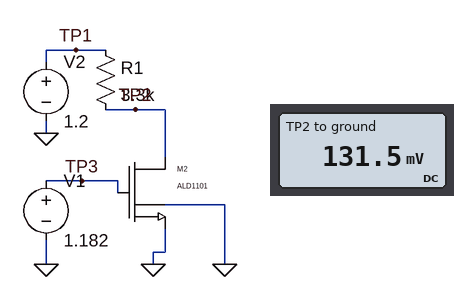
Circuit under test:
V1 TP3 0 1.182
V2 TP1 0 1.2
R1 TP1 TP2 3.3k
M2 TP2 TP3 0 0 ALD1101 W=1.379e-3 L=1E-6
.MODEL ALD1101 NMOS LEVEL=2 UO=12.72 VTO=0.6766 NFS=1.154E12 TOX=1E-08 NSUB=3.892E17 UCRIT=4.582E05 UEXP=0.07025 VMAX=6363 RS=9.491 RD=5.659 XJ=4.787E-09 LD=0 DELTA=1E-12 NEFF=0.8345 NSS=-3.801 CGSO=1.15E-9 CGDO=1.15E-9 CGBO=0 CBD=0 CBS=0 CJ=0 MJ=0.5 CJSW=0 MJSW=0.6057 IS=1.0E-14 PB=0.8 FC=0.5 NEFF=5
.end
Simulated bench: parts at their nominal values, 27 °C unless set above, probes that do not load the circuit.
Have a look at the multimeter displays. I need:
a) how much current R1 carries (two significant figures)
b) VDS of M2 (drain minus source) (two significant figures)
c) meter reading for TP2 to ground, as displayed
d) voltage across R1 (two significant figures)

320 µA
130 mV
131.5 mV
1.1 V
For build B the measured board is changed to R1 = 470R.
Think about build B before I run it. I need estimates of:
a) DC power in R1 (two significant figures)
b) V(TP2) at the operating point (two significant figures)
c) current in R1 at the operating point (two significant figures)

140 µW
940 mV
550 µA
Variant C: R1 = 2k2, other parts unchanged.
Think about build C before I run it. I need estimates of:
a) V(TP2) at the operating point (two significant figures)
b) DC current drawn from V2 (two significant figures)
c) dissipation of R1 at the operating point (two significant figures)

210 mV
450 µA
440 µW
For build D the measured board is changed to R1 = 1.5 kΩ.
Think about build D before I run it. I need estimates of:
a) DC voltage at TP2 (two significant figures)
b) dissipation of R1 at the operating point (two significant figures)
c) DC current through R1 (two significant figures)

390 mV
430 µW
540 µA
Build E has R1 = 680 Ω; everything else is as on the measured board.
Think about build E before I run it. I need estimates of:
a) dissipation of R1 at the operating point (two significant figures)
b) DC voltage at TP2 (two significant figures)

200 µW
830 mV
